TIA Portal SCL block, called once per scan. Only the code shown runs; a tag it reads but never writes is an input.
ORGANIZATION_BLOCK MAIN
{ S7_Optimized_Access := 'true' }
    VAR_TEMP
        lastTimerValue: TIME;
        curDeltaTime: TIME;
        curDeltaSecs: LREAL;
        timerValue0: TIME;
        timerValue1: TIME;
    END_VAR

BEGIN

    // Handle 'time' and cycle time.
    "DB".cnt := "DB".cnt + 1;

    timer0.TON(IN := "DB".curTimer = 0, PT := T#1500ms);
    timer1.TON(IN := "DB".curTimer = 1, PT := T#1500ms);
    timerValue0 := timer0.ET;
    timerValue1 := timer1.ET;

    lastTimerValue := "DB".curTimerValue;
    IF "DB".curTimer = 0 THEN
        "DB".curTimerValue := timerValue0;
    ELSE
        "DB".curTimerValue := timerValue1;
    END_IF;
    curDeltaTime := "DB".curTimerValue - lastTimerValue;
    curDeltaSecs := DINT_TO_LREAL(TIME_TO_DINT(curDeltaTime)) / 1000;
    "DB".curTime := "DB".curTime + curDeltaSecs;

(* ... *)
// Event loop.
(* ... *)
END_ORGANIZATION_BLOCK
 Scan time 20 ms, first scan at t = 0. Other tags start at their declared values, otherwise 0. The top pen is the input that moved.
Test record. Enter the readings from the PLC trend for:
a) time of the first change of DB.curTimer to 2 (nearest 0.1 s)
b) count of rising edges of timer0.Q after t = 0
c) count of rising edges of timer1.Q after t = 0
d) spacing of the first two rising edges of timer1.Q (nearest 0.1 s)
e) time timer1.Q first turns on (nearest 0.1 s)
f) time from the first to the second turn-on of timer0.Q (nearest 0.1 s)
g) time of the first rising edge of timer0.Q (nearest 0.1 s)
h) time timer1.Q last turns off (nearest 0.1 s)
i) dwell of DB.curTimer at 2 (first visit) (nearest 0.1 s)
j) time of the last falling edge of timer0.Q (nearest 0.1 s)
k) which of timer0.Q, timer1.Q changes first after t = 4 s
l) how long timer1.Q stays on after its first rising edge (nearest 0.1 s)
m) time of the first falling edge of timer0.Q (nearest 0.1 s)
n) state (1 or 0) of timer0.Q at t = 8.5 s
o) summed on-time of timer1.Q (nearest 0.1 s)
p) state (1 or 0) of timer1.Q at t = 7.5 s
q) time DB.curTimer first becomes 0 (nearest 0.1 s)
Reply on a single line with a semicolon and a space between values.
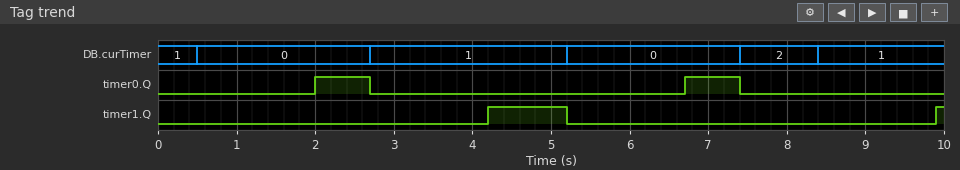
7.4 s; 2; 2; 5.7 s; 4.2 s; 4.7 s; 2.0 s; 5.2 s; 1.0 s; 7.4 s; timer1.Q; 1.0 s; 2.7 s; 0; 1.1 s; 0; 0.5 s
